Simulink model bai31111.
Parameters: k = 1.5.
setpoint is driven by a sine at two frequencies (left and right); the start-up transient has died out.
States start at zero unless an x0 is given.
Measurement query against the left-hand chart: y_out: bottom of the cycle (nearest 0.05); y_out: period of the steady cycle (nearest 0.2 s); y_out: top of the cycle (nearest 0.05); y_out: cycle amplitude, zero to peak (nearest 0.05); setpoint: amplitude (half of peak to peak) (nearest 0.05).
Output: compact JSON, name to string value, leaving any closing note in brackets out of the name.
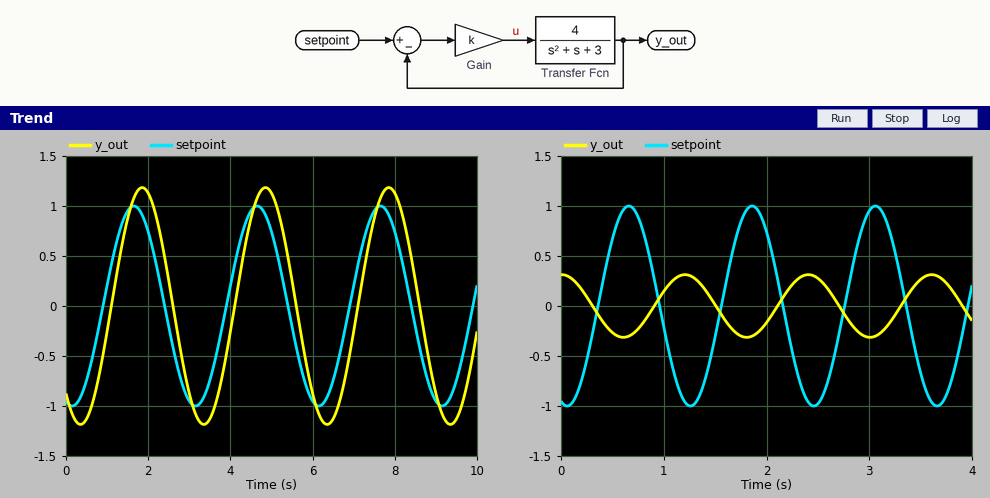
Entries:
{"y_out: bottom of the cycle": "-1.20", "y_out: period of the steady cycle": "3.0 s", "y_out: top of the cycle": "1.20", "y_out: cycle amplitude, zero to peak": "1.20", "setpoint: amplitude (half of peak to peak)": "1.00"}
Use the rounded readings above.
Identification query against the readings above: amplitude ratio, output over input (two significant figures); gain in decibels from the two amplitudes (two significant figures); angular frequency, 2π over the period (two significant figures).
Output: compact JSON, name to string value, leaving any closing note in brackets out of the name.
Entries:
{"amplitude ratio, output over input": "1.2", "gain in decibels from the two amplitudes": "1.6 dB", "angular frequency, 2π over the period": "2.1 rad/s"}
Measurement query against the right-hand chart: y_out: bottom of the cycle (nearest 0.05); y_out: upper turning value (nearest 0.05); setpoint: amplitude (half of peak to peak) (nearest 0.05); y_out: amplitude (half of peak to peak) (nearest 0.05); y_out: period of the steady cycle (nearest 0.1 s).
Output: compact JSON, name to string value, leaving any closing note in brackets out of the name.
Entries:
{"y_out: bottom of the cycle": "-0.30", "y_out: upper turning value": "0.30", "setpoint: amplitude (half of peak to peak)": "1.00", "y_out: amplitude (half of peak to peak)": "0.30", "y_out: period of the steady cycle": "1.2 s"}
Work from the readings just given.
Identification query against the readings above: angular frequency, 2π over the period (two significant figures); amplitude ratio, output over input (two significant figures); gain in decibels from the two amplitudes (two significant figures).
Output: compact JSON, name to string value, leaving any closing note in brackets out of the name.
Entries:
{"angular frequency, 2π over the period": "5.2 rad/s", "amplitude ratio, output over input": "0.30", "gain in decibels from the two amplitudes": "-10 dB"}
